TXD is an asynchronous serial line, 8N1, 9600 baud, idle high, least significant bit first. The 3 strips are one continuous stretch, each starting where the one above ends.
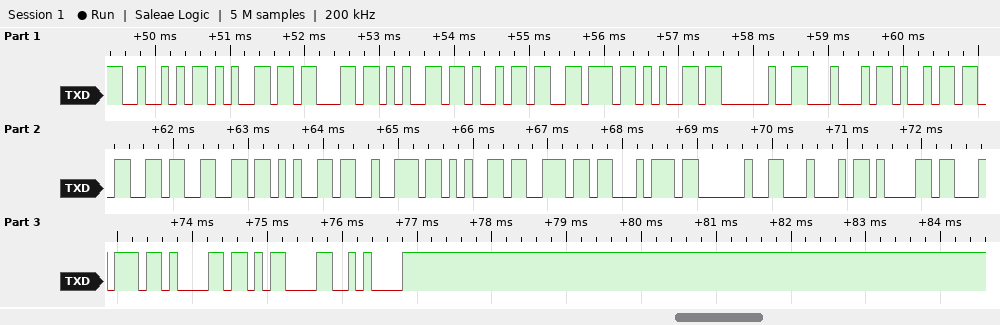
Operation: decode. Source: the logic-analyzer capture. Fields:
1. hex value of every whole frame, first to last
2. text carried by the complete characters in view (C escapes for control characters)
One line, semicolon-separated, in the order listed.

52 65 63 65 69 76 65 20 44 69 66 66 65 72 65 6E 74 20 44 61 74 61 0D 0A; "Receive Different Data\r\n"
